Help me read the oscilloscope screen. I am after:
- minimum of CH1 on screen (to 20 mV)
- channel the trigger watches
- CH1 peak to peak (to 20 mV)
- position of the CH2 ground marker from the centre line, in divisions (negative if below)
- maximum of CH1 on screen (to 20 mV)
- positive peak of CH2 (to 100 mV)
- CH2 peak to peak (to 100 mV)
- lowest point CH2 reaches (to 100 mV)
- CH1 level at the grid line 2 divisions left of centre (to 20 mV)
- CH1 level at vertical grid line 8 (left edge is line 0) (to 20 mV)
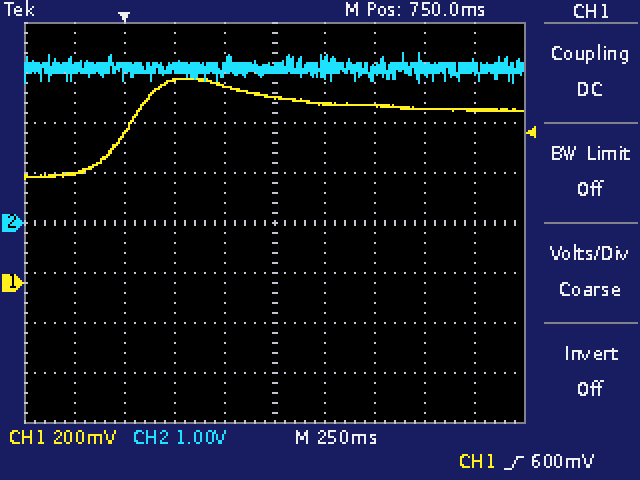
420 mV
CH1
400 mV
0.0 div
820 mV
3.4 V
600 mV
2.8 V
820 mV
700 mV
